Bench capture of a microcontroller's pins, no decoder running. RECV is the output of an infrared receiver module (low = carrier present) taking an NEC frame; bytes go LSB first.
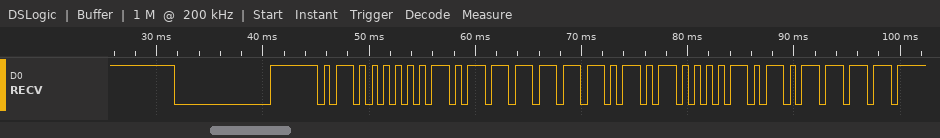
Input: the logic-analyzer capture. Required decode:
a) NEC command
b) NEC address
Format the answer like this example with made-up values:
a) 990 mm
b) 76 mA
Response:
a) 0x0A
b) 0x02
